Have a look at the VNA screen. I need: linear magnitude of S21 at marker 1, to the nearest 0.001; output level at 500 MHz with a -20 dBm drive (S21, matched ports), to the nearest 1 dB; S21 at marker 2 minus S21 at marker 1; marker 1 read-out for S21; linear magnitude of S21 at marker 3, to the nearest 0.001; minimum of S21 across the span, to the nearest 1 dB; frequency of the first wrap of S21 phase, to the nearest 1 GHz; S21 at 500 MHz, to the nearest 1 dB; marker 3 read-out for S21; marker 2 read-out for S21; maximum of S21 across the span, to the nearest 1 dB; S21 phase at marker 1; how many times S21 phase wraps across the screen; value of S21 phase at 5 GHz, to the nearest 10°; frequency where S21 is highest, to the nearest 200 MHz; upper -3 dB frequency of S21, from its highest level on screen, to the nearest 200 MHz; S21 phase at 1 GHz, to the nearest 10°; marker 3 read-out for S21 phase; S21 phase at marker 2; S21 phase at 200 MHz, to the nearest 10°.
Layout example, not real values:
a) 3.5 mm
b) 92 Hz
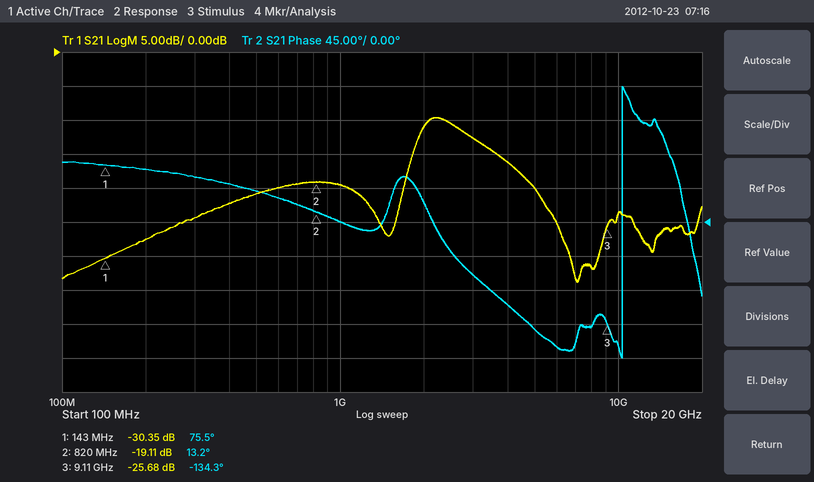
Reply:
a) 0.030
b) -41 dBm
c) 11.24 dB
d) -30.35 dB
e) 0.052
f) -34 dB
g) 10 GHz
h) -21 dB
i) -25.68 dB
j) -19.11 dB
k) -10 dB
l) 75.5°
m) 1
n) -140°
o) 2.2 GHz
p) 3.0 GHz
q) 0°
r) -134.3°
s) 13.2°
t) 70°
